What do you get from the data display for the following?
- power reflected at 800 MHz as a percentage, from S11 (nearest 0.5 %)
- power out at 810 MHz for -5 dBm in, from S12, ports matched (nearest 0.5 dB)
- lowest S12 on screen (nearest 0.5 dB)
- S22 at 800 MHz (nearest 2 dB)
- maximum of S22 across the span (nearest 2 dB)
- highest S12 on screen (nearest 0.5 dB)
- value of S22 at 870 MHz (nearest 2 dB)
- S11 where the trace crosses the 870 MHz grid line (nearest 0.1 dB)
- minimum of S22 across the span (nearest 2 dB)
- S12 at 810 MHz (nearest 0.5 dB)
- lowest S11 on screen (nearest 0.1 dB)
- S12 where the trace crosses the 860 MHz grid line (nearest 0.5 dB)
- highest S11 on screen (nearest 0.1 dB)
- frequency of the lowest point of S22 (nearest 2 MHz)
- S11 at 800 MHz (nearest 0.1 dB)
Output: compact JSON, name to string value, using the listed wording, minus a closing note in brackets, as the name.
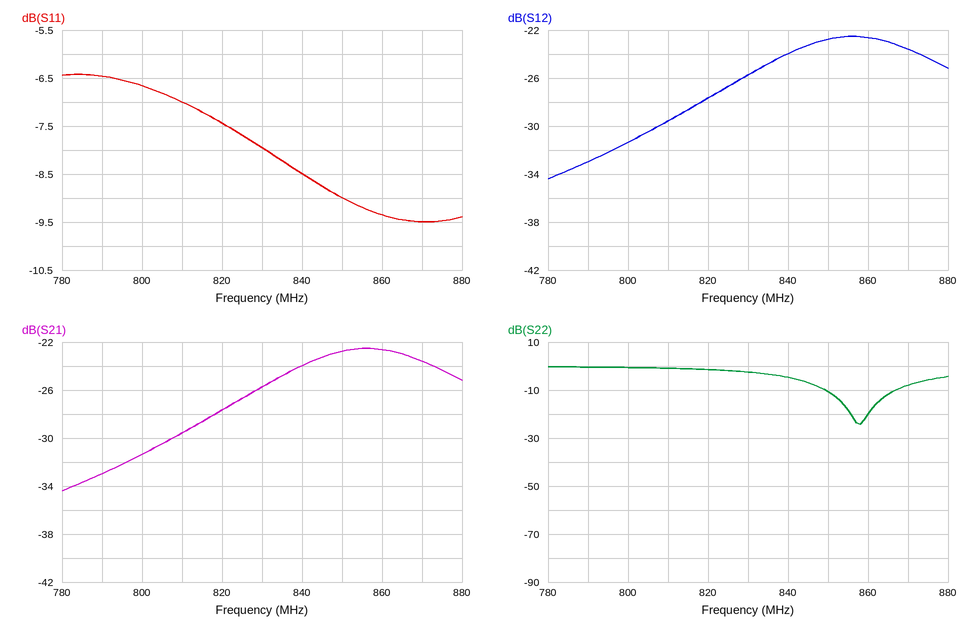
{"power reflected at 800 MHz as a percentage, from S11": "21.5 %", "power out at 810 MHz for -5 dBm in, from S12, ports matched": "-34.5 dBm", "lowest S12 on screen": "-34.5 dB", "S22 at 800 MHz": "0 dB", "maximum of S22 across the span": "0 dB", "highest S12 on screen": "-22.5 dB", "value of S22 at 870 MHz": "-8 dB", "S11 where the trace crosses the 870 MHz grid line": "-9.5 dB", "minimum of S22 across the span": "-24 dB", "S12 at 810 MHz": "-29.5 dB", "lowest S11 on screen": "-9.5 dB", "S12 where the trace crosses the 860 MHz grid line": "-22.5 dB", "highest S11 on screen": "-6.4 dB", "frequency of the lowest point of S22": "858 MHz", "S11 at 800 MHz": "-6.7 dB"}
